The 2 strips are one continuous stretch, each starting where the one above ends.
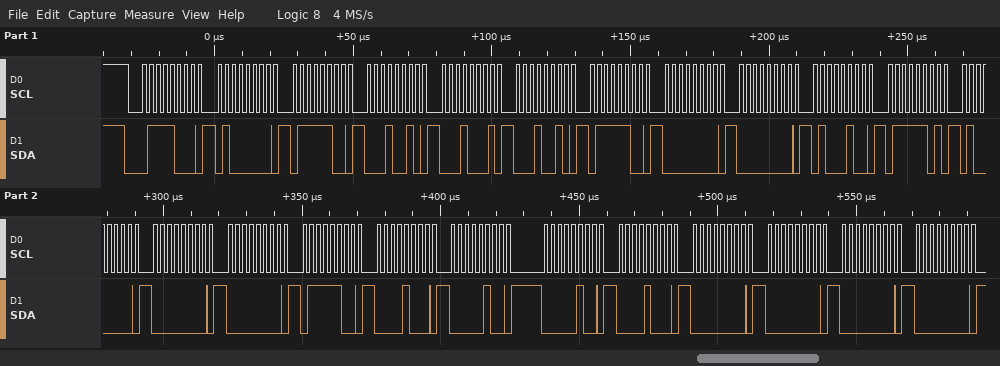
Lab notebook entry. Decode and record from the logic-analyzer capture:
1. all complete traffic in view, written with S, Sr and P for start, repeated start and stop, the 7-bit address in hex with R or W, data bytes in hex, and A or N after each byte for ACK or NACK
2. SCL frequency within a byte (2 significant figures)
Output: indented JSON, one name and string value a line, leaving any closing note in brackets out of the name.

{
  "all complete traffic in view, written with S, Sr and P for start, repeated start and stop, the 7-bit address in hex with R or W, data bytes in hex, and A or N after each byte for ACK or NACK": "S 3CW A 40 A 7C A 12 A 11 A 12 A 7C A 00 A 00 A 44 A 7D A 40 A 00 A 00 A 7C A 08 A 04 A 04 A 08 A 00 A 00 A 00 A 00 A",
  "SCL frequency within a byte": "400 kHz"
}
